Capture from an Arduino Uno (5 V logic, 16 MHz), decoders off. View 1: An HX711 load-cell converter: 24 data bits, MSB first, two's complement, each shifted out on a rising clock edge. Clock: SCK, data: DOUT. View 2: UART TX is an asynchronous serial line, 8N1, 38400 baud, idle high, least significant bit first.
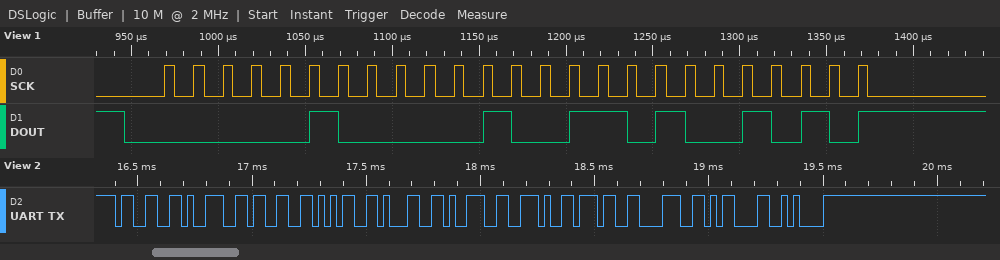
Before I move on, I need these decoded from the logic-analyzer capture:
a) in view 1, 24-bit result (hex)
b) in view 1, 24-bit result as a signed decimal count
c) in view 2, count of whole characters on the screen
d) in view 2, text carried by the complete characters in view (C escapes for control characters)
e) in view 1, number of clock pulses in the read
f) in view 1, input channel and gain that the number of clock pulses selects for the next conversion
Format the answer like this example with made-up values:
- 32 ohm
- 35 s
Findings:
- 0x04134A
- 267082
- 11
- "393519.78\r\n"
- 25
- channel A, gain 128
